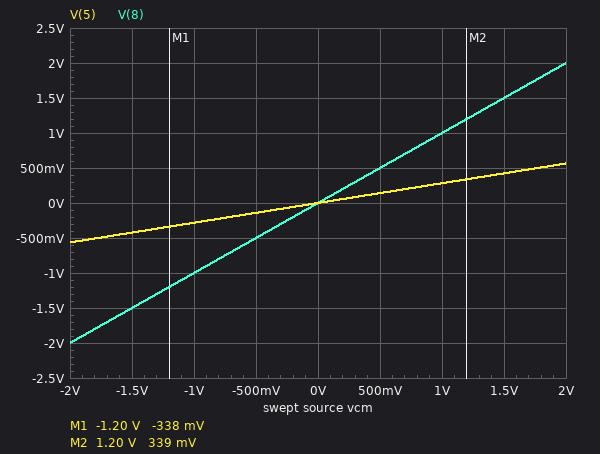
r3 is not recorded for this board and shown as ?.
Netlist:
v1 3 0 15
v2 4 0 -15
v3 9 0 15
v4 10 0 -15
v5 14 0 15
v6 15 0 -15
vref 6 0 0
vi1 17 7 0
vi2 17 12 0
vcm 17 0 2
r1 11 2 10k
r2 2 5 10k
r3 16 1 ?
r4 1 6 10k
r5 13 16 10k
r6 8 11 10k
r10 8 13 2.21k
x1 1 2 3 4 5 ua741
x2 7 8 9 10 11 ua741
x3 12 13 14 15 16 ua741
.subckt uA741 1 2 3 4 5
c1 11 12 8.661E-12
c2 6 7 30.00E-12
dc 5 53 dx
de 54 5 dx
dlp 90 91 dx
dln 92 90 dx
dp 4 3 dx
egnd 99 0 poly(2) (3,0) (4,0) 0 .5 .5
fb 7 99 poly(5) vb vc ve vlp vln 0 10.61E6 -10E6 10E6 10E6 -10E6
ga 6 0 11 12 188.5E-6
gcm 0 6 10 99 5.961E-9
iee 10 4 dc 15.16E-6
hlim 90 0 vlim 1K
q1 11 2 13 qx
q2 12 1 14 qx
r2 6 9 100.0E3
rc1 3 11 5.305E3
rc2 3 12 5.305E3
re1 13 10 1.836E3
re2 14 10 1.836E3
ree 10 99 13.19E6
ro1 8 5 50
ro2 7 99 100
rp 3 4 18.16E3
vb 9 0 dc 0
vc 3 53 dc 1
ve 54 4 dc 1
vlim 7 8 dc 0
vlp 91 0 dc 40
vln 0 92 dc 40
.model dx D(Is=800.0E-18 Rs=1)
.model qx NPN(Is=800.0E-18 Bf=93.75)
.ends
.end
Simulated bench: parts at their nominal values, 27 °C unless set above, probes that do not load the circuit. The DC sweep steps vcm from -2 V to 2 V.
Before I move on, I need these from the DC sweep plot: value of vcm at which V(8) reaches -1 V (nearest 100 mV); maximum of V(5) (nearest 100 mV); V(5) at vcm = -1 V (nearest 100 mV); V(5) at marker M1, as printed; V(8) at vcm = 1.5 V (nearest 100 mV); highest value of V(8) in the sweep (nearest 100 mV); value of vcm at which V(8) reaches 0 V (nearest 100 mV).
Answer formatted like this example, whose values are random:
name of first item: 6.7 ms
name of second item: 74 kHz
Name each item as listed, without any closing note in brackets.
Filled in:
value of vcm at which V(8) reaches -1 V: -1.0 V
maximum of V(5): 600 mV
V(5) at vcm = -1 V: -300 mV
V(5) at marker M1, as printed: -338 mV
V(8) at vcm = 1.5 V: 1.5 V
highest value of V(8) in the sweep: 2.0 V
value of vcm at which V(8) reaches 0 V: 0 V
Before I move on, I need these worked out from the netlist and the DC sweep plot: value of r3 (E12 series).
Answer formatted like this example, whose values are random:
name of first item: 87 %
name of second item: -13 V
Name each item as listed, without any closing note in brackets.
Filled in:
value of r3: 5.6 kΩ
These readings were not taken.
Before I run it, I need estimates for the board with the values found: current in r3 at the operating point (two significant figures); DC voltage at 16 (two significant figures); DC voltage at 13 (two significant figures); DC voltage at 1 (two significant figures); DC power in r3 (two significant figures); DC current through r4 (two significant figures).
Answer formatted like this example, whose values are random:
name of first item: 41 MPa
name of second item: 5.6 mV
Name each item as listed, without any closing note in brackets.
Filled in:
current in r3 at the operating point: 130 µA
DC voltage at 16: 2.0 V
DC voltage at 13: 2.0 V
DC voltage at 1: 1.3 V
DC power in r3: 92 µW
DC current through r4: 130 µA
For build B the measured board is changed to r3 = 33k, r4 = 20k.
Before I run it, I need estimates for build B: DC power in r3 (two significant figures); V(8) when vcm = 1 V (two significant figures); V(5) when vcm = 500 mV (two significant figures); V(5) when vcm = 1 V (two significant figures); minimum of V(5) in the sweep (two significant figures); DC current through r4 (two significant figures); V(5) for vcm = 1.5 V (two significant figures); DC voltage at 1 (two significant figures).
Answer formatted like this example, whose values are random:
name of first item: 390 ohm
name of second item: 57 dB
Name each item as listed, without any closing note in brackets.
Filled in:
DC power in r3: 47 µW
V(8) when vcm = 1 V: 1.0 V
V(5) when vcm = 500 mV: -120 mV
V(5) when vcm = 1 V: -250 mV
minimum of V(5) in the sweep: -490 mV
DC current through r4: 38 µA
V(5) for vcm = 1.5 V: -370 mV
DC voltage at 1: 750 mV
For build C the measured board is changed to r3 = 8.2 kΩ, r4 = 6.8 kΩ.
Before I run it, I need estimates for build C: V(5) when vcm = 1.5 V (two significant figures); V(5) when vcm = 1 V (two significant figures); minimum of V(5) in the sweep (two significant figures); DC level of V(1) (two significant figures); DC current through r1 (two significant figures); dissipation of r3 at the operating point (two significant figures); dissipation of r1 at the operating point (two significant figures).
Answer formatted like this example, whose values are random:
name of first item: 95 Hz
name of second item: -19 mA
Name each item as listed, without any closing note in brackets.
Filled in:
V(5) when vcm = 1.5 V: -140 mV
V(5) when vcm = 1 V: -93 mV
minimum of V(5) in the sweep: -190 mV
DC level of V(1): 910 mV
DC current through r1: 110 µA
dissipation of r3 at the operating point: 150 µW
dissipation of r1 at the operating point: 120 µW
